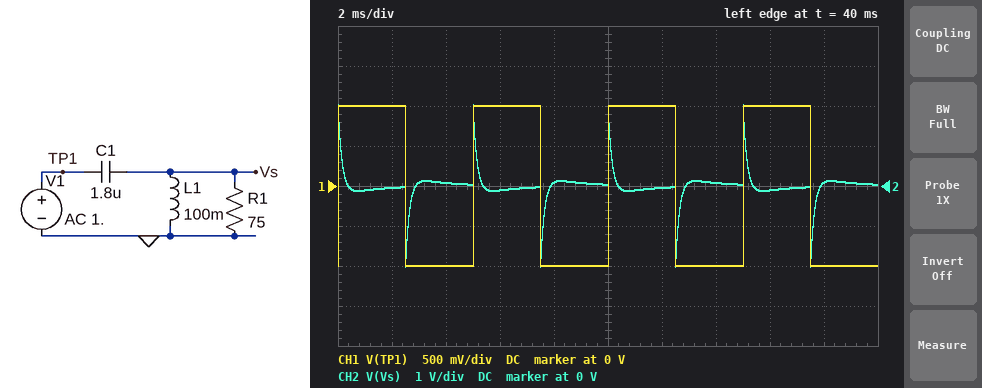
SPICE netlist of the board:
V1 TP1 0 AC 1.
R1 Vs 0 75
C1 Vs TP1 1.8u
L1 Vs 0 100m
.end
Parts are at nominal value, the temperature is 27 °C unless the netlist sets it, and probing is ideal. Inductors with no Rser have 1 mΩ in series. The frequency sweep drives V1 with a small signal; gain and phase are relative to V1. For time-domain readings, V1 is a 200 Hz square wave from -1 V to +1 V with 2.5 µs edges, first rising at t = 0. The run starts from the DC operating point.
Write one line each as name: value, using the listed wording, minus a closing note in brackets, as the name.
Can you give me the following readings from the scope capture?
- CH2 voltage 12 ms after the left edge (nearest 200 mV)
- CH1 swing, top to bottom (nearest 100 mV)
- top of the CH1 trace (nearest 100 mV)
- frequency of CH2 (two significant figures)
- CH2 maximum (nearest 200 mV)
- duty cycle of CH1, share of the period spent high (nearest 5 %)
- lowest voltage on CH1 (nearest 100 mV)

CH2 voltage 12 ms after the left edge: 0 V
CH1 swing, top to bottom: 2.0 V
top of the CH1 trace: 1.0 V
frequency of CH2: 200 Hz
CH2 maximum: 2.0 V
duty cycle of CH1, share of the period spent high: 50 %
lowest voltage on CH1: -1.0 V
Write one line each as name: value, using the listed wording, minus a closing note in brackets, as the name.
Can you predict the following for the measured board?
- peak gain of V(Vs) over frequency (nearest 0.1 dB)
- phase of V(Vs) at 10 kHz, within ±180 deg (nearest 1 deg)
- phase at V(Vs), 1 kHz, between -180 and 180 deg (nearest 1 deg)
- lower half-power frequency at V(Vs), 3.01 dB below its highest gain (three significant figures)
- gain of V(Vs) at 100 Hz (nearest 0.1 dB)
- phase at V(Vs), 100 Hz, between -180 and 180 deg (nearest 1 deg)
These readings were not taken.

peak gain of V(Vs) over frequency: 0 dB
phase of V(Vs) at 10 kHz, within ±180 deg: 7 deg
phase at V(Vs), 1 kHz, between -180 and 180 deg: 54 deg
lower half-power frequency at V(Vs), 3.01 dB below its highest gain: 1.06 kHz
gain of V(Vs) at 100 Hz: -24.9 dB
phase at V(Vs), 100 Hz, between -180 and 180 deg: 138 deg
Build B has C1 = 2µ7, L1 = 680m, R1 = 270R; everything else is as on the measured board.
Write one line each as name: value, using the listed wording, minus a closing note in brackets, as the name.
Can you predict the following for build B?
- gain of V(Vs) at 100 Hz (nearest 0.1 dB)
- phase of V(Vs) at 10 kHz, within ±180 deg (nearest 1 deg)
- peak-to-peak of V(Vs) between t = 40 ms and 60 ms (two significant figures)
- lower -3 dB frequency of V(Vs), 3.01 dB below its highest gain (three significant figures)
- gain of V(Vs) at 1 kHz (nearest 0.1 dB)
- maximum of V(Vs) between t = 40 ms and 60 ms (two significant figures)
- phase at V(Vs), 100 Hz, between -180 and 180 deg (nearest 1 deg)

gain of V(Vs) at 100 Hz: -6.9 dB
phase of V(Vs) at 10 kHz, within ±180 deg: 1 deg
peak-to-peak of V(Vs) between t = 40 ms and 60 ms: 4.3 V
lower -3 dB frequency of V(Vs), 3.01 dB below its highest gain: 165 Hz
gain of V(Vs) at 1 kHz: -0.1 dB
maximum of V(Vs) between t = 40 ms and 60 ms: 2.2 V
phase at V(Vs), 100 Hz, between -180 and 180 deg: 100 deg
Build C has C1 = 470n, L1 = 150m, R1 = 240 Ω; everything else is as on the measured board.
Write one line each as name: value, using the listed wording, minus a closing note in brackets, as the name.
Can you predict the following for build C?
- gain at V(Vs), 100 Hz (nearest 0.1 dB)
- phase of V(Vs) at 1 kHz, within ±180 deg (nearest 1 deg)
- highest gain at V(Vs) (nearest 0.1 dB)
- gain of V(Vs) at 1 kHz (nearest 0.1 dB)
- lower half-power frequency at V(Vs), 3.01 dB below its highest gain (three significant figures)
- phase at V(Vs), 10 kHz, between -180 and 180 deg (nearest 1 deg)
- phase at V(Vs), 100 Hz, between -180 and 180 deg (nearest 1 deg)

gain at V(Vs), 100 Hz: -31.5 dB
phase of V(Vs) at 1 kHz, within ±180 deg: 66 deg
highest gain at V(Vs): 0 dB
gain of V(Vs) at 1 kHz: -3.8 dB
lower half-power frequency at V(Vs), 3.01 dB below its highest gain: 1.17 kHz
phase at V(Vs), 10 kHz, between -180 and 180 deg: 8 deg
phase at V(Vs), 100 Hz, between -180 and 180 deg: 158 deg
